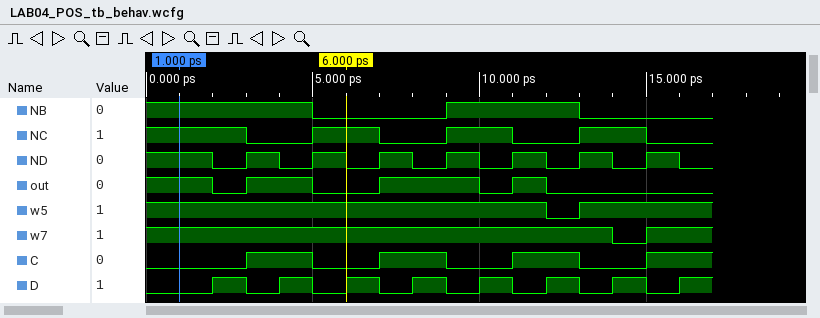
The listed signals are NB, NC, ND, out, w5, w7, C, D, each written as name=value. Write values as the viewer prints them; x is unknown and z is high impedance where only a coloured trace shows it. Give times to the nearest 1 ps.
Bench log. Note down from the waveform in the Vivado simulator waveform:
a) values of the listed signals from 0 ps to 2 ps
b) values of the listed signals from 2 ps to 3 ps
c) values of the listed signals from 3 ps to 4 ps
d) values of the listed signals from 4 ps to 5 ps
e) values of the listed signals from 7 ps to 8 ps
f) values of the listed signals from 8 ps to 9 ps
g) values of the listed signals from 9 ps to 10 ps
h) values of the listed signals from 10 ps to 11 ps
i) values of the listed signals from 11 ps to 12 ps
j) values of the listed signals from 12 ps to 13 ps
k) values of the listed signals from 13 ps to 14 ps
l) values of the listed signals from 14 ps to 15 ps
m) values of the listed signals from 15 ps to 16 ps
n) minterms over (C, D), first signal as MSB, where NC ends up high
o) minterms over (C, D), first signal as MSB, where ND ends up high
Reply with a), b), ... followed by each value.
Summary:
a) NB=1, NC=1, ND=1, out=1, w5=1, w7=1, C=0, D=0
b) NB=1, NC=1, ND=0, out=0, w5=1, w7=1, C=0, D=1
c) NB=1, NC=0, ND=1, out=1, w5=1, w7=1, C=1, D=0
d) NB=1, NC=0, ND=0, out=1, w5=1, w7=1, C=1, D=1
e) NB=0, NC=0, ND=1, out=1, w5=1, w7=1, C=1, D=0
f) NB=0, NC=0, ND=0, out=1, w5=1, w7=1, C=1, D=1
g) NB=1, NC=1, ND=1, out=1, w5=1, w7=1, C=0, D=0
h) NB=1, NC=1, ND=0, out=0, w5=1, w7=1, C=0, D=1
i) NB=1, NC=0, ND=1, out=1, w5=1, w7=1, C=1, D=0
j) NB=1, NC=0, ND=0, out=0, w5=0, w7=1, C=1, D=1
k) NB=0, NC=1, ND=1, out=0, w5=1, w7=1, C=0, D=0
l) NB=0, NC=1, ND=0, out=0, w5=1, w7=0, C=0, D=1
m) NB=0, NC=0, ND=1, out=0, w5=1, w7=1, C=1, D=0
n) 0, 1
o) 0, 2
